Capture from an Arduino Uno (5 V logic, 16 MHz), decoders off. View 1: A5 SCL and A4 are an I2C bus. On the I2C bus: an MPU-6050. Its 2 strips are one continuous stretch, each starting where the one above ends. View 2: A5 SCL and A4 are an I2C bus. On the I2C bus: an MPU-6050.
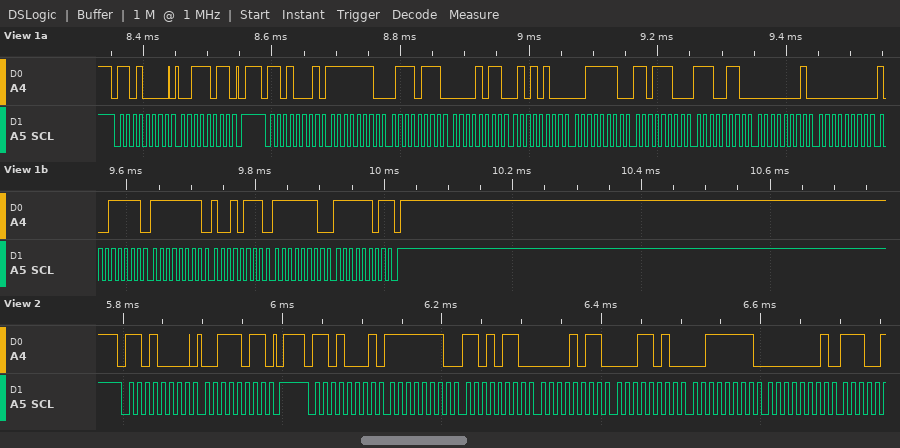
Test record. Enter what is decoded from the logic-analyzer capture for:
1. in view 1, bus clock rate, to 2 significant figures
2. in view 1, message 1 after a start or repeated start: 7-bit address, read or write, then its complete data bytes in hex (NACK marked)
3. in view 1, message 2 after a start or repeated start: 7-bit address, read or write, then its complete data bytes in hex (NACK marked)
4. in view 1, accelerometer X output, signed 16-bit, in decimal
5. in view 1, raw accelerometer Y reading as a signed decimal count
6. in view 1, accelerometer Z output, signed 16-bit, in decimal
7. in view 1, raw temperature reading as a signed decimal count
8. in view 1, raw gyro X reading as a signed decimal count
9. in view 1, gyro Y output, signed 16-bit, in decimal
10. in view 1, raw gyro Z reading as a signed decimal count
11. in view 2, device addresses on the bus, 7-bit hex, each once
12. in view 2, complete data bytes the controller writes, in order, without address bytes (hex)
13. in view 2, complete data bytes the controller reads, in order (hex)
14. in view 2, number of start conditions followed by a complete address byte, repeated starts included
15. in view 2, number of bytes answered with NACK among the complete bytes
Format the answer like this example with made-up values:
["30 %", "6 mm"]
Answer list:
["100 kHz", "0x68 write: 3B", "0x68 read: FE 77 0B 54 3E DC E6 01 00 9F FF 97 FE FD NACK", "-393", "2900", "16092", "-6655", "159", "-105", "-259", "0x68", "3B", "FE D6 0B 1A 3F 01", "2", "0"]
